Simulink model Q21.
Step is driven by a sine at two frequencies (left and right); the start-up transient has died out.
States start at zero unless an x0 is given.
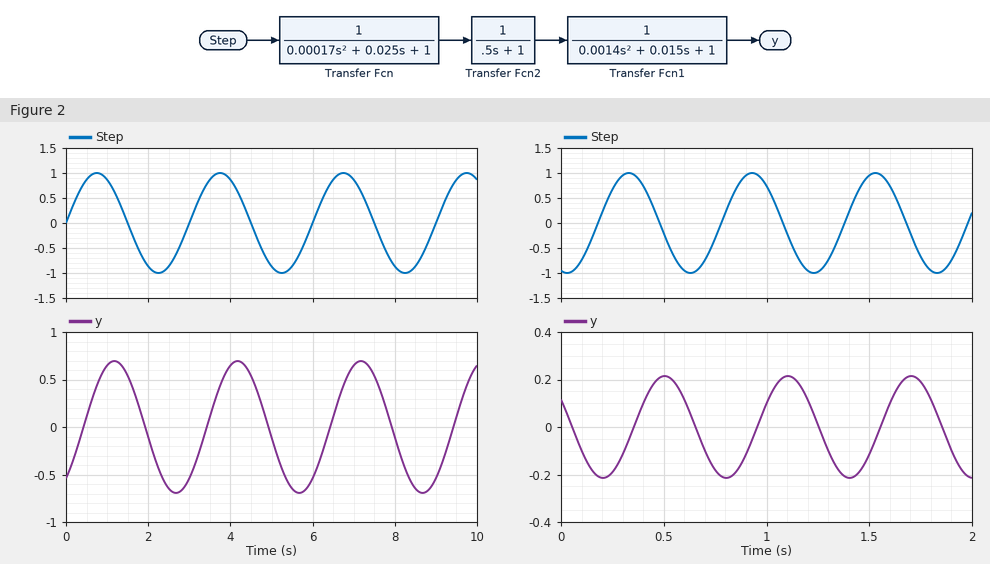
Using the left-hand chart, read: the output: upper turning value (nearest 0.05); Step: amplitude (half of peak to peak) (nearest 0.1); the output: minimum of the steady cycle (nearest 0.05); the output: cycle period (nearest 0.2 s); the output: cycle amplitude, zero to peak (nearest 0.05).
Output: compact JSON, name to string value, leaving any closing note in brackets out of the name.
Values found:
{"the output: upper turning value": "0.70", "Step: amplitude (half of peak to peak)": "1.0", "the output: minimum of the steady cycle": "-0.70", "the output: cycle period": "3.0 s", "the output: cycle amplitude, zero to peak": "0.70"}
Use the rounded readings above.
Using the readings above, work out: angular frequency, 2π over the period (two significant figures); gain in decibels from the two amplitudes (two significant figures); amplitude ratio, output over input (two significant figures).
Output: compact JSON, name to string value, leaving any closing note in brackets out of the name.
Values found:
{"angular frequency, 2π over the period": "2.1 rad/s", "gain in decibels from the two amplitudes": "-3.1 dB", "amplitude ratio, output over input": "0.70"}
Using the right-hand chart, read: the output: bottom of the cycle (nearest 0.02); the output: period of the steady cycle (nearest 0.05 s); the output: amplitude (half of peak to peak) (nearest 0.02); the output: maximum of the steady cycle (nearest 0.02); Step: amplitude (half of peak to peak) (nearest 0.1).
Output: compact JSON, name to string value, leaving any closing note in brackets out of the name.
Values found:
{"the output: bottom of the cycle": "-0.22", "the output: period of the steady cycle": "0.60 s", "the output: amplitude (half of peak to peak)": "0.22", "the output: maximum of the steady cycle": "0.22", "Step: amplitude (half of peak to peak)": "1.0"}
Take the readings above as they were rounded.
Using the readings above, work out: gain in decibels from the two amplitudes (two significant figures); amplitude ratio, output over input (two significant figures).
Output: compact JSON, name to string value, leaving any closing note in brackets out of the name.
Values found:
{"gain in decibels from the two amplitudes": "-13 dB", "amplitude ratio, output over input": "0.22"}
